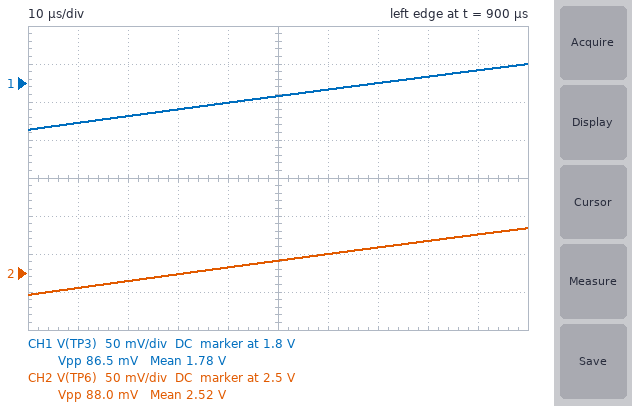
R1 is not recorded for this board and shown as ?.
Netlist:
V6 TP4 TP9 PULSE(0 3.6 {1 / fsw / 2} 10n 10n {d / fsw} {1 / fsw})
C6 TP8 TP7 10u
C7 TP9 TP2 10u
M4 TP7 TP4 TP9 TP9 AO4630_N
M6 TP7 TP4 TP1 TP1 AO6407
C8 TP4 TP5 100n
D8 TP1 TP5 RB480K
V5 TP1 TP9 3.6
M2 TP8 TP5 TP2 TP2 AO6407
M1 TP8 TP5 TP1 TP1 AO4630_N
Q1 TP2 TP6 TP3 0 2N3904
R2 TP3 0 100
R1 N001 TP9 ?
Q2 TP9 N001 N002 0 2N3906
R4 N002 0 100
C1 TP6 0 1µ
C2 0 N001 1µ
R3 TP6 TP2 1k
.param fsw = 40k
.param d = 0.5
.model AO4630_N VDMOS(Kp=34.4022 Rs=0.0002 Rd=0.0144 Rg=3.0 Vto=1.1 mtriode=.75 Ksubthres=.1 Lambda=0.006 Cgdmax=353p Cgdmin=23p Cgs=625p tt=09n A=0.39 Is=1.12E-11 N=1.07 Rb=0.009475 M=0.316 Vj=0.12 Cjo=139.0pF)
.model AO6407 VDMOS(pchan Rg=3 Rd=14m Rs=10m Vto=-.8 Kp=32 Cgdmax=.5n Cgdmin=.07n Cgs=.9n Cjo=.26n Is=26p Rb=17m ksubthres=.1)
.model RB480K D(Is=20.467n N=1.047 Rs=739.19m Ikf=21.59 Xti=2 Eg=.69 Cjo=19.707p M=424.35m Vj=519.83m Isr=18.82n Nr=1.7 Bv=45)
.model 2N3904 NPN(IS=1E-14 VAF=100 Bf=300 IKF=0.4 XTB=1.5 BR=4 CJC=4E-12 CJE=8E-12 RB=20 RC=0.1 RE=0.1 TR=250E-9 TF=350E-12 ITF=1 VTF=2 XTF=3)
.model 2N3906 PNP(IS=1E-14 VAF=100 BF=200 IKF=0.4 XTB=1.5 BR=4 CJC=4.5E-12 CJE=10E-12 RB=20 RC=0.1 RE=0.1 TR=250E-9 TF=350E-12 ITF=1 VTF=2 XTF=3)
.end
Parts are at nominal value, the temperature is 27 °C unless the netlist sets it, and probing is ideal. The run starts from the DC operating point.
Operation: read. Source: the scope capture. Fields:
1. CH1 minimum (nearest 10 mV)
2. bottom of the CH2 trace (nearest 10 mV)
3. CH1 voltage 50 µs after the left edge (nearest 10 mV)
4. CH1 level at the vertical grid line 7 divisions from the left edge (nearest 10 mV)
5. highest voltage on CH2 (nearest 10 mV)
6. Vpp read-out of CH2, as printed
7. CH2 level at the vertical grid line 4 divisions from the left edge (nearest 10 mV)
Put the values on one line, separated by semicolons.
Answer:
1.74 V; 2.47 V; 1.78 V; 1.80 V; 2.56 V; 88.0 mV; 2.51 V
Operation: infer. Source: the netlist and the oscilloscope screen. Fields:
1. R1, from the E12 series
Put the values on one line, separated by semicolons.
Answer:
1.2 kΩ
